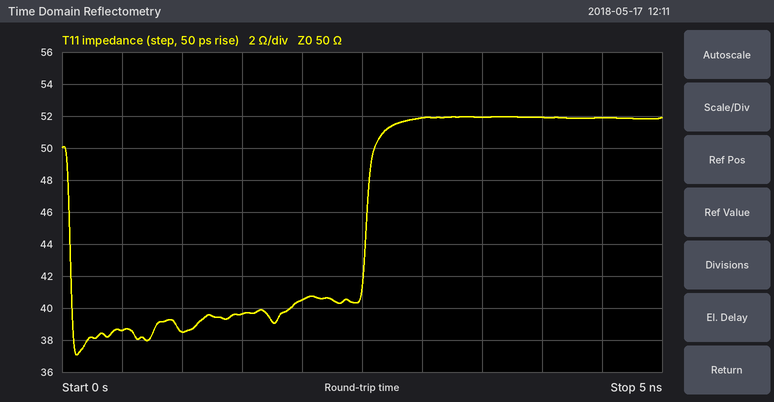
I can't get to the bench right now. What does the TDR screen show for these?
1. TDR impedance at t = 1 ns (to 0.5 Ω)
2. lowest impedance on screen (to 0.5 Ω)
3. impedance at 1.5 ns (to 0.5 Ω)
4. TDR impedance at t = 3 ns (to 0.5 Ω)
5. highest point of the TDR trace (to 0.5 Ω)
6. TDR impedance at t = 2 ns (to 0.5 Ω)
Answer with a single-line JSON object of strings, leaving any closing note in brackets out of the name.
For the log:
{"TDR impedance at t = 1 ns": "38.5 Ω", "lowest impedance on screen": "37.0 Ω", "impedance at 1.5 ns": "39.5 Ω", "TDR impedance at t = 3 ns": "52.0 Ω", "highest point of the TDR trace": "52.0 Ω", "TDR impedance at t = 2 ns": "40.5 Ω"}
